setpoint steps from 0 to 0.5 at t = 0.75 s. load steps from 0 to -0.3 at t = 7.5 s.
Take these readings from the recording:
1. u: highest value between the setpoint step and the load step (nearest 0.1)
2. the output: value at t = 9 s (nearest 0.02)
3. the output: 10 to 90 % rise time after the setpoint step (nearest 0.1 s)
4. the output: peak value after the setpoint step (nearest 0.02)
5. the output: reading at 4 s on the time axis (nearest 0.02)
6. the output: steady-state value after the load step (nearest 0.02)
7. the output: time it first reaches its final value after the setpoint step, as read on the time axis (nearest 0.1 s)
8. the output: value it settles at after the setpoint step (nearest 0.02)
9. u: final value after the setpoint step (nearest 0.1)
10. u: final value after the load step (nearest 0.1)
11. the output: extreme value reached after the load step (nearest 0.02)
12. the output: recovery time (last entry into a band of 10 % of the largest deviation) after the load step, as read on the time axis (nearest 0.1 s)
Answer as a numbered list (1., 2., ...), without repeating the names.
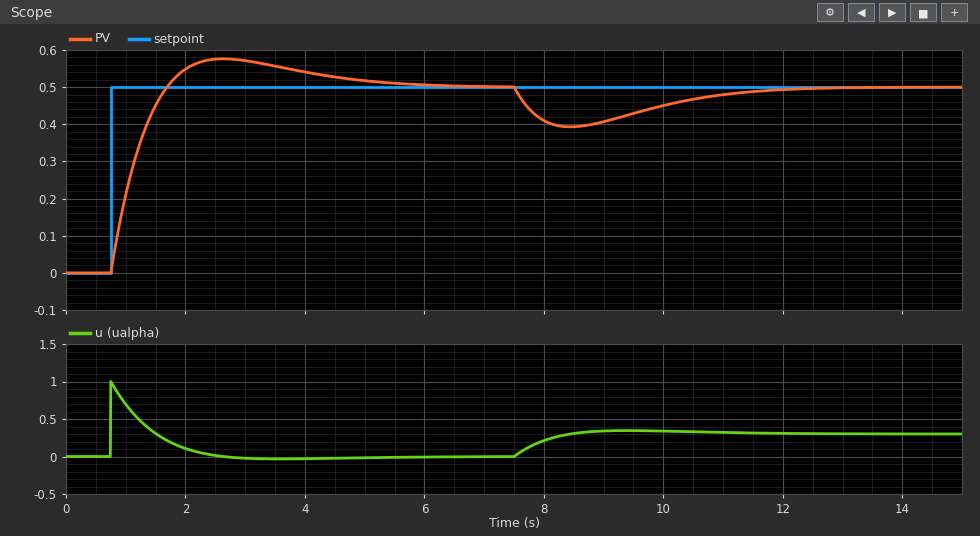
1. 1.0
2. 0.40
3. 0.7 s
4. 0.58
5. 0.54
6. 0.50
7. 1.7 s
8. 0.50
9. 0.0
10. 0.3
11. 0.40
12. 11.6 s
